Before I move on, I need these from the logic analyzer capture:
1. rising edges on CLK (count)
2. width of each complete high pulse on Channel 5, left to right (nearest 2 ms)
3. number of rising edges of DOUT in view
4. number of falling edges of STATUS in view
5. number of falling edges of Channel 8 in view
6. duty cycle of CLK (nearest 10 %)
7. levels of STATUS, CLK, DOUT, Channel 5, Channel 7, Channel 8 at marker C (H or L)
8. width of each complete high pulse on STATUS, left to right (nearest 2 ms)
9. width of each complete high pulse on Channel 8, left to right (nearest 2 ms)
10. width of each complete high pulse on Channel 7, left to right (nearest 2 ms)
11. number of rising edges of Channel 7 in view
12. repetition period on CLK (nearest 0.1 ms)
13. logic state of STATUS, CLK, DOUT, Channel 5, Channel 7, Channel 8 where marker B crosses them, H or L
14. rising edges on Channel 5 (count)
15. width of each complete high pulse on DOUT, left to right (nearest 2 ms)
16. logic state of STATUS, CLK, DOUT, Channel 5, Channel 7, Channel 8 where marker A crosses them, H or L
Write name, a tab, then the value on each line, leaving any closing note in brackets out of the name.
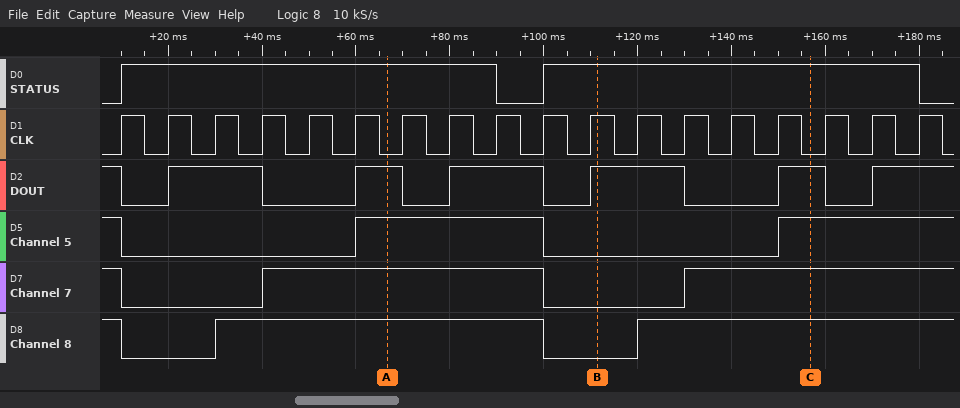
rising edges on CLK	18
width of each complete high pulse on Channel 5, left to right	40 ms
number of rising edges of DOUT in view	6
number of falling edges of STATUS in view	2
number of falling edges of Channel 8 in view	2
duty cycle of CLK	50 %
levels of STATUS, CLK, DOUT, Channel 5, Channel 7, Channel 8 at marker C	STATUS=H, CLK=L, DOUT=H, Channel 5=H, Channel 7=H, Channel 8=H
width of each complete high pulse on STATUS, left to right	80 ms, 80 ms
width of each complete high pulse on Channel 8, left to right	70 ms
width of each complete high pulse on Channel 7, left to right	60 ms
number of rising edges of Channel 7 in view	2
repetition period on CLK	10 ms
logic state of STATUS, CLK, DOUT, Channel 5, Channel 7, Channel 8 where marker B crosses them, H or L	STATUS=H, CLK=H, DOUT=H, Channel 5=L, Channel 7=L, Channel 8=L
rising edges on Channel 5	2
width of each complete high pulse on DOUT, left to right	20 ms, 10 ms, 20 ms, 20 ms, 10 ms
logic state of STATUS, CLK, DOUT, Channel 5, Channel 7, Channel 8 where marker A crosses them, H or L	STATUS=H, CLK=L, DOUT=H, Channel 5=H, Channel 7=H, Channel 8=H
